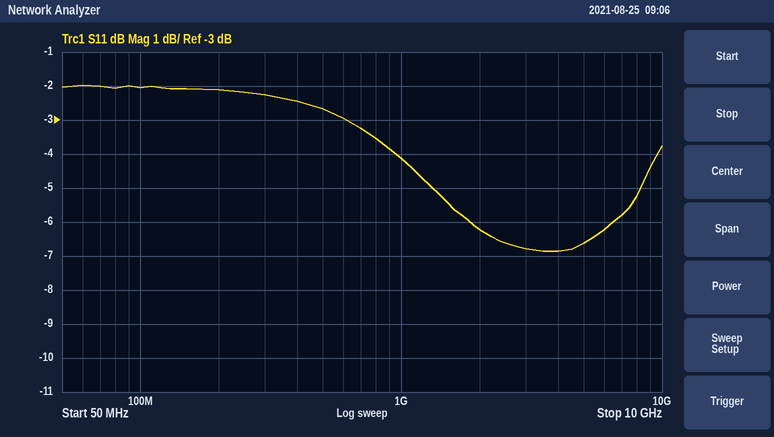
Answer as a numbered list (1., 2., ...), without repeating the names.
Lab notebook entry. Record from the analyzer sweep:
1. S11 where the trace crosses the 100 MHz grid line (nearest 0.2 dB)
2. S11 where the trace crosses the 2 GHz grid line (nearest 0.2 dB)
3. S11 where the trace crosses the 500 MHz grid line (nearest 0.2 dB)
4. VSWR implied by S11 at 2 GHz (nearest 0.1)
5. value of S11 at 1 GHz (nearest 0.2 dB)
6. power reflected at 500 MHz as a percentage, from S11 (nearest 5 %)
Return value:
1. -2.0 dB
2. -6.2 dB
3. -2.6 dB
4. 2.9
5. -4.2 dB
6. 55 %
